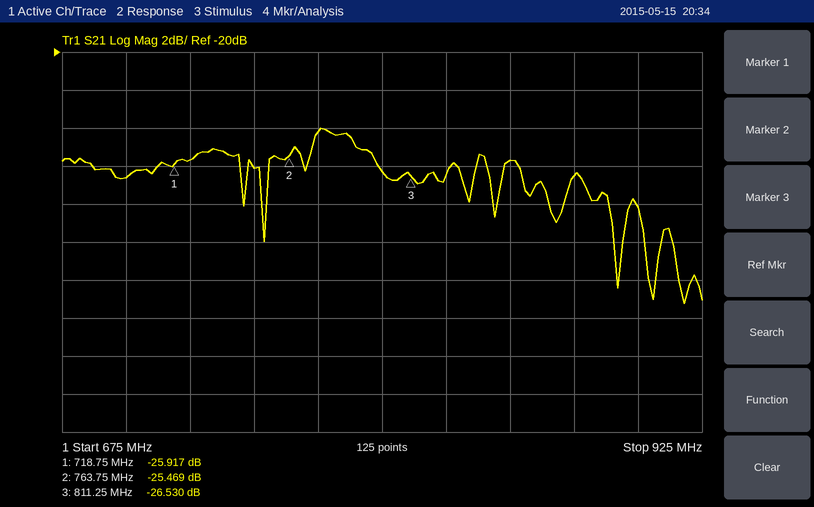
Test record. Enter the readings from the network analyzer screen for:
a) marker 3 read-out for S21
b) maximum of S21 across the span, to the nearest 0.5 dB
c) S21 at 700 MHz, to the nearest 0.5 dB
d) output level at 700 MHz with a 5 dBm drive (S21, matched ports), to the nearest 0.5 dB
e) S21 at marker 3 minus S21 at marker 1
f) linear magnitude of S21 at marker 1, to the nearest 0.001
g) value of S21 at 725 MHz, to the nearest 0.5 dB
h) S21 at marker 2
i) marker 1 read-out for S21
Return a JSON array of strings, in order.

["-26.530 dB", "-24.0 dB", "-26.5 dB", "-21.5 dBm", "-0.613 dB", "0.051", "-25.5 dB", "-25.469 dB", "-25.917 dB"]
